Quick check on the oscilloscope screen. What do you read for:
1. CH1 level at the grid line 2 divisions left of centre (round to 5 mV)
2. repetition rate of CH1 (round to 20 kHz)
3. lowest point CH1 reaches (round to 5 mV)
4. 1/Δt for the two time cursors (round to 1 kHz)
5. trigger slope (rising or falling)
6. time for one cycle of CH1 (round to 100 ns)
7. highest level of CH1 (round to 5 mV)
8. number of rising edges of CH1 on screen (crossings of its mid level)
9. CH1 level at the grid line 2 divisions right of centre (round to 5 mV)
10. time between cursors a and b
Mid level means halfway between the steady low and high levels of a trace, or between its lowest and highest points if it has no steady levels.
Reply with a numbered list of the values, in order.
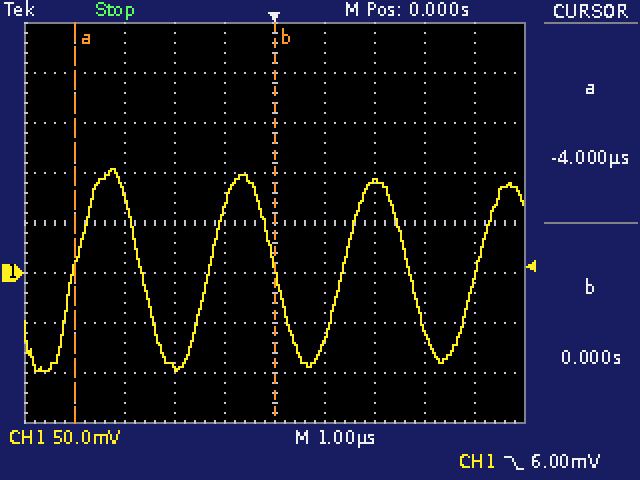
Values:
1. -95 mV
2. 380 kHz
3. -100 mV
4. 250 kHz
5. falling
6. 2.7 µs
7. 105 mV
8. 4
9. 90 mV
10. 4.0 µs
